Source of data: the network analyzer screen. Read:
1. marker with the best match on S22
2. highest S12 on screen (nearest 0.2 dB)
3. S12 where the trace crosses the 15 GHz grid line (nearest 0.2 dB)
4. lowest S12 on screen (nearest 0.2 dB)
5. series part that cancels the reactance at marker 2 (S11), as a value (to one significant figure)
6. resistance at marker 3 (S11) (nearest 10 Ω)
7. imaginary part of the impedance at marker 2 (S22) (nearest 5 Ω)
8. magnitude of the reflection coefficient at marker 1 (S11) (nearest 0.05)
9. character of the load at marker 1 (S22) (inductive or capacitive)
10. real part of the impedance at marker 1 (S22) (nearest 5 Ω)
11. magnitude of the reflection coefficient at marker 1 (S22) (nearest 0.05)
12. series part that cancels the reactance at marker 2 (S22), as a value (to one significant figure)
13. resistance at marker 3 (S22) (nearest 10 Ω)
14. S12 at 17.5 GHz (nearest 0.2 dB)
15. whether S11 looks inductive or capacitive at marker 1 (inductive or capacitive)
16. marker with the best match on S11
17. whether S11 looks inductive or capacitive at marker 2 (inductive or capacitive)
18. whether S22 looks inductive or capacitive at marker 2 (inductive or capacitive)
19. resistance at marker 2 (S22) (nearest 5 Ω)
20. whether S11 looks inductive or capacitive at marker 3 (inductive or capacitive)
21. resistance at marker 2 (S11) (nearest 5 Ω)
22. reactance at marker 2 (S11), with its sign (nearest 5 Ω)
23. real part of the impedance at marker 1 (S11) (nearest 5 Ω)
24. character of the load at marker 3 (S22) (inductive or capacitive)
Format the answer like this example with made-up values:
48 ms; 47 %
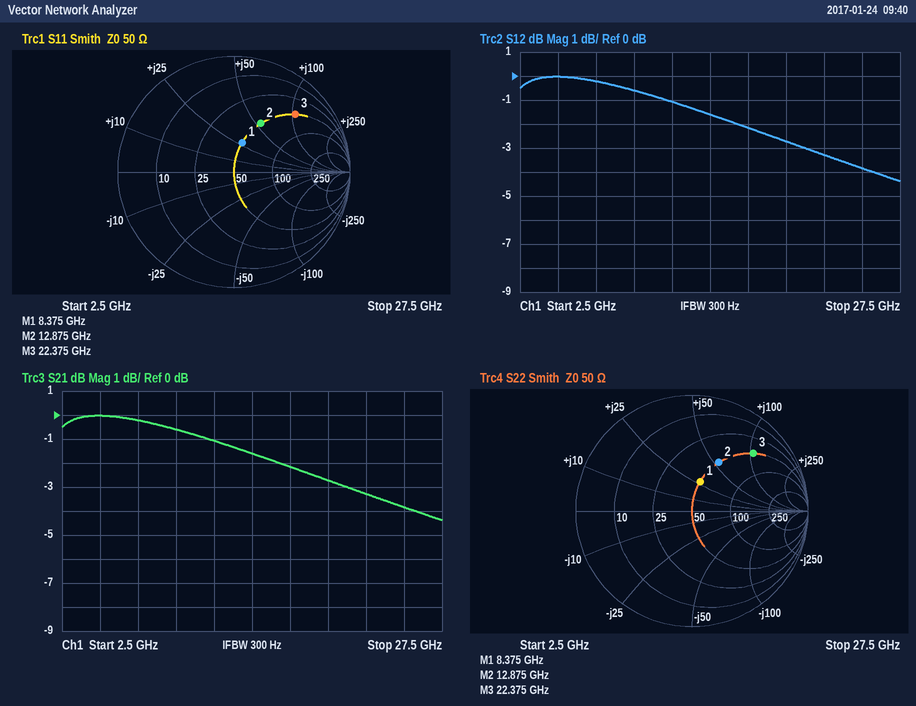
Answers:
marker 1; 0.0 dB; -1.6 dB; -4.4 dB; 200 fF; 50 Ω; +55 Ω; 0.25; inductive; 50 Ω; 0.25; 200 fF; 50 Ω; -2.2 dB; inductive; marker 1; inductive; inductive; 50 Ω; inductive; 50 Ω; +55 Ω; 50 Ω; inductive
